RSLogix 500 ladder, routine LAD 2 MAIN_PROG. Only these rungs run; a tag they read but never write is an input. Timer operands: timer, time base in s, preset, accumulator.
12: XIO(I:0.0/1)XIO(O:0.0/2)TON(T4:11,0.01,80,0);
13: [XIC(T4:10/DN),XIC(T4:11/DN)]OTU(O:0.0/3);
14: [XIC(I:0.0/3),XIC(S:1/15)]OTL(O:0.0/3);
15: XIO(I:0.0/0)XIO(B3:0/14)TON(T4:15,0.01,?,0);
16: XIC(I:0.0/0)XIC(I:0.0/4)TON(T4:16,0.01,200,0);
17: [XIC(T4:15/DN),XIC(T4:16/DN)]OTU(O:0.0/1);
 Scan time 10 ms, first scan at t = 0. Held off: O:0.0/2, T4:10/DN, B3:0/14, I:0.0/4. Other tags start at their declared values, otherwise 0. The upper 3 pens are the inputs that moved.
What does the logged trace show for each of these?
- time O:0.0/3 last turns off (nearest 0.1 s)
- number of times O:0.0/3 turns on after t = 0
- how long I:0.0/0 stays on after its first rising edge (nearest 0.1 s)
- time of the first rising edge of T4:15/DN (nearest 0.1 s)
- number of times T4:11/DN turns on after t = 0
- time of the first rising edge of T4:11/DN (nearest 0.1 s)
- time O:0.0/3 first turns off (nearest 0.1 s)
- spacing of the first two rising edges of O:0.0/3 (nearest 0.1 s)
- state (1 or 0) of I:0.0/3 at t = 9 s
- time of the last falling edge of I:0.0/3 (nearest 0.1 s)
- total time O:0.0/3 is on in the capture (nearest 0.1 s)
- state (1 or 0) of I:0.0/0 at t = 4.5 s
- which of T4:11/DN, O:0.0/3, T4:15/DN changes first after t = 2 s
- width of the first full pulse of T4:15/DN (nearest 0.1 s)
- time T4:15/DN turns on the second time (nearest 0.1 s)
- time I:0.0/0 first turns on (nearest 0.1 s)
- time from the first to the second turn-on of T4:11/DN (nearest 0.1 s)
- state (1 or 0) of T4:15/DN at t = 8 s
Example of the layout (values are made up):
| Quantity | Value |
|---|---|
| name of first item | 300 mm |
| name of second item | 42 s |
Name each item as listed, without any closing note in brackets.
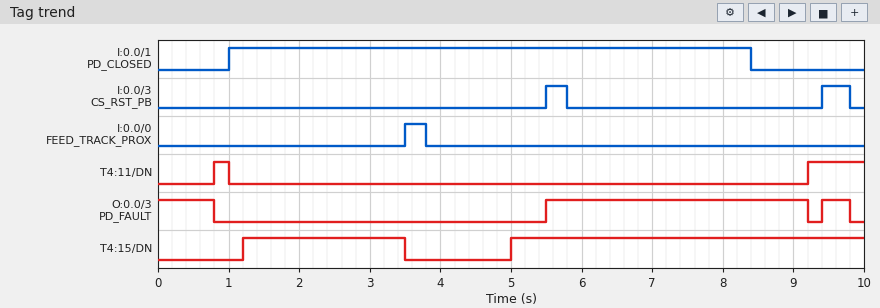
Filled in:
| Quantity | Value |
|---|---|
| time O:0.0/3 last turns off | 9.8 s |
| number of times O:0.0/3 turns on after t = 0 | 2 |
| how long I:0.0/0 stays on after its first rising edge | 0.3 s |
| time of the first rising edge of T4:15/DN | 1.2 s |
| number of times T4:11/DN turns on after t = 0 | 2 |
| time of the first rising edge of T4:11/DN | 0.8 s |
| time O:0.0/3 first turns off | 0.8 s |
| spacing of the first two rising edges of O:0.0/3 | 3.9 s |
| state (1 or 0) of I:0.0/3 at t = 9 s | 0 |
| time of the last falling edge of I:0.0/3 | 9.8 s |
| total time O:0.0/3 is on in the capture | 4.9 s |
| state (1 or 0) of I:0.0/0 at t = 4.5 s | 0 |
| which of T4:11/DN, O:0.0/3, T4:15/DN changes first after t = 2 s | T4:15/DN |
| width of the first full pulse of T4:15/DN | 2.3 s |
| time T4:15/DN turns on the second time | 5.0 s |
| time I:0.0/0 first turns on | 3.5 s |
| time from the first to the second turn-on of T4:11/DN | 8.4 s |
| state (1 or 0) of T4:15/DN at t = 8 s | 1 |
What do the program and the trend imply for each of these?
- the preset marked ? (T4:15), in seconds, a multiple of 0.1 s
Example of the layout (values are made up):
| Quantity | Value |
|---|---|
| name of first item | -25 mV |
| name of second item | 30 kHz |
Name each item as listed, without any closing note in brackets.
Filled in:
| Quantity | Value |
|---|---|
| the preset marked ? (T4:15), in seconds, a multiple of 0.1 s | 1.2 s |
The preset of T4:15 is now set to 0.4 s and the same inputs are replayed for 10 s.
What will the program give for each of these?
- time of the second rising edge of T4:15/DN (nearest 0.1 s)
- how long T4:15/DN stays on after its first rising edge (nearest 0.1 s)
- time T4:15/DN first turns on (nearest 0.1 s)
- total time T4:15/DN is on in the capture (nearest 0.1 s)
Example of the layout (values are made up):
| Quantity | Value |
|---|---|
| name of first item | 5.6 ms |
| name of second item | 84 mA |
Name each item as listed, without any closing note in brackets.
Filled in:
| Quantity | Value |
|---|---|
| time of the second rising edge of T4:15/DN | 4.2 s |
| how long T4:15/DN stays on after its first rising edge | 3.1 s |
| time T4:15/DN first turns on | 0.4 s |
| total time T4:15/DN is on in the capture | 8.9 s |
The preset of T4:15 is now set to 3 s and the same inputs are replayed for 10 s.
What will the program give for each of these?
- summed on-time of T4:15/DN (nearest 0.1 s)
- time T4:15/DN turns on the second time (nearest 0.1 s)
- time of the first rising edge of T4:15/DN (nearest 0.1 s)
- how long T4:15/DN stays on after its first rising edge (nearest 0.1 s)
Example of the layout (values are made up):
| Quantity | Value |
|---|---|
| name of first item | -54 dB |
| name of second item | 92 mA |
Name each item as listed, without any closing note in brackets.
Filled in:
| Quantity | Value |
|---|---|
| summed on-time of T4:15/DN | 3.7 s |
| time T4:15/DN turns on the second time | 6.8 s |
| time of the first rising edge of T4:15/DN | 3.0 s |
| how long T4:15/DN stays on after its first rising edge | 0.5 s |
